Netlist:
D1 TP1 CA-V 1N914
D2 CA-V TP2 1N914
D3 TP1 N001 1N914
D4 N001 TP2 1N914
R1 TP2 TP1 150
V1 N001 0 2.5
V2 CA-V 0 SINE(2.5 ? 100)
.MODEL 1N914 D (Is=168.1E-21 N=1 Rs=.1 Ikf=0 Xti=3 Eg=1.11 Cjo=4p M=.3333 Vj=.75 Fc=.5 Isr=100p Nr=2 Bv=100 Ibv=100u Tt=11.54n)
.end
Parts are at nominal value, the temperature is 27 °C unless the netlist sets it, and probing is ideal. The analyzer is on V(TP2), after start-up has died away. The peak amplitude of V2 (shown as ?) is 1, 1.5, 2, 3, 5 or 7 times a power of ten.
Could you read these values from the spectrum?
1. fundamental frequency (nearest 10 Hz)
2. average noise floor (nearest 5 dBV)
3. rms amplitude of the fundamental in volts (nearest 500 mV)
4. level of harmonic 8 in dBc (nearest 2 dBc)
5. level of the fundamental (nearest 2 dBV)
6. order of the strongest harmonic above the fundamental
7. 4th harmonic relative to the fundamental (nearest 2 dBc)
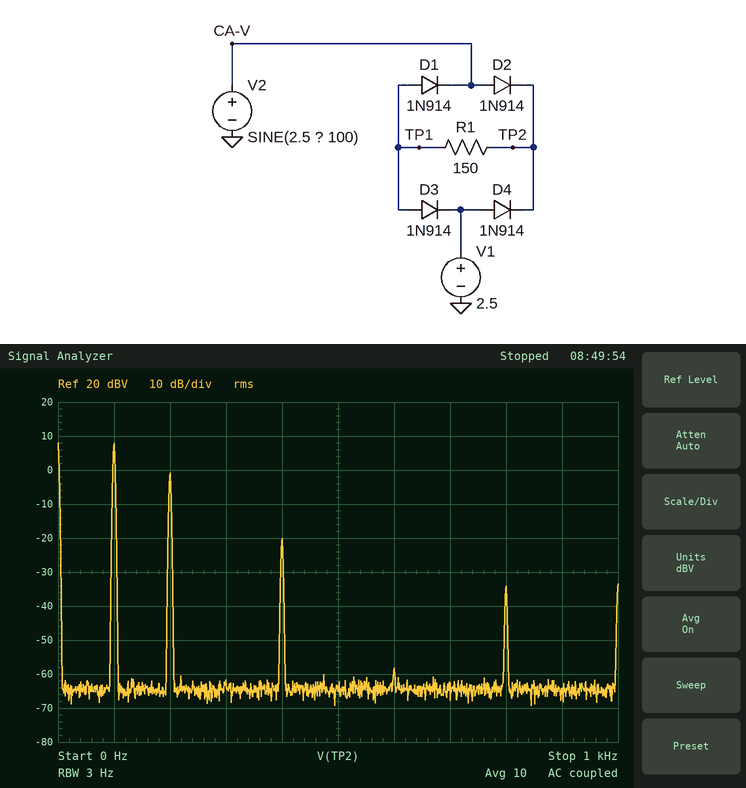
100 Hz
-65 dBV
2.5 V
-42 dBc
8 dBV
2
-28 dBc
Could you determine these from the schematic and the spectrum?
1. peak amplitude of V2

7 V
